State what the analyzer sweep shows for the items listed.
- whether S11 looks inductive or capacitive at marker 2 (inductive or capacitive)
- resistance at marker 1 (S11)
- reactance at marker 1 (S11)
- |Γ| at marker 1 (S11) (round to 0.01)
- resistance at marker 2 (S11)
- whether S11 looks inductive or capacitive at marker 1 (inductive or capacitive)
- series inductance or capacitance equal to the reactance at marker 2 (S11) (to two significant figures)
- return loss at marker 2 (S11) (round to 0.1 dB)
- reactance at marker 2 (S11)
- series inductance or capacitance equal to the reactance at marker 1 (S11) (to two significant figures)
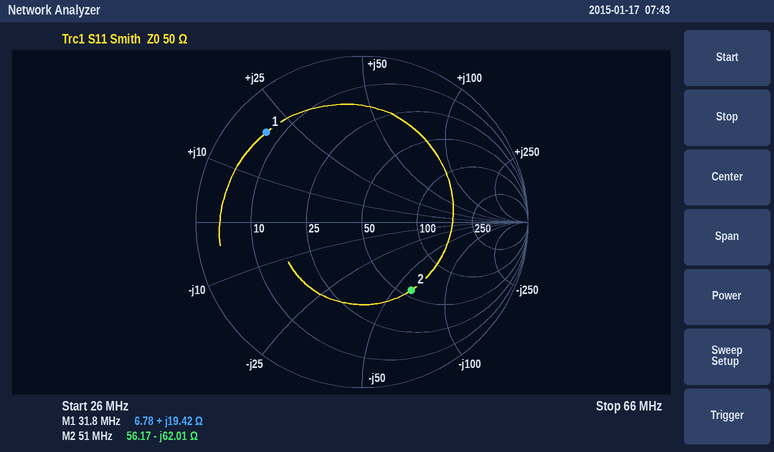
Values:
capacitive
6.78 Ω
+19.42 Ω
0.79
56.17 Ω
inductive
50 pF
5.9 dB
-62.01 Ω
97 nH
